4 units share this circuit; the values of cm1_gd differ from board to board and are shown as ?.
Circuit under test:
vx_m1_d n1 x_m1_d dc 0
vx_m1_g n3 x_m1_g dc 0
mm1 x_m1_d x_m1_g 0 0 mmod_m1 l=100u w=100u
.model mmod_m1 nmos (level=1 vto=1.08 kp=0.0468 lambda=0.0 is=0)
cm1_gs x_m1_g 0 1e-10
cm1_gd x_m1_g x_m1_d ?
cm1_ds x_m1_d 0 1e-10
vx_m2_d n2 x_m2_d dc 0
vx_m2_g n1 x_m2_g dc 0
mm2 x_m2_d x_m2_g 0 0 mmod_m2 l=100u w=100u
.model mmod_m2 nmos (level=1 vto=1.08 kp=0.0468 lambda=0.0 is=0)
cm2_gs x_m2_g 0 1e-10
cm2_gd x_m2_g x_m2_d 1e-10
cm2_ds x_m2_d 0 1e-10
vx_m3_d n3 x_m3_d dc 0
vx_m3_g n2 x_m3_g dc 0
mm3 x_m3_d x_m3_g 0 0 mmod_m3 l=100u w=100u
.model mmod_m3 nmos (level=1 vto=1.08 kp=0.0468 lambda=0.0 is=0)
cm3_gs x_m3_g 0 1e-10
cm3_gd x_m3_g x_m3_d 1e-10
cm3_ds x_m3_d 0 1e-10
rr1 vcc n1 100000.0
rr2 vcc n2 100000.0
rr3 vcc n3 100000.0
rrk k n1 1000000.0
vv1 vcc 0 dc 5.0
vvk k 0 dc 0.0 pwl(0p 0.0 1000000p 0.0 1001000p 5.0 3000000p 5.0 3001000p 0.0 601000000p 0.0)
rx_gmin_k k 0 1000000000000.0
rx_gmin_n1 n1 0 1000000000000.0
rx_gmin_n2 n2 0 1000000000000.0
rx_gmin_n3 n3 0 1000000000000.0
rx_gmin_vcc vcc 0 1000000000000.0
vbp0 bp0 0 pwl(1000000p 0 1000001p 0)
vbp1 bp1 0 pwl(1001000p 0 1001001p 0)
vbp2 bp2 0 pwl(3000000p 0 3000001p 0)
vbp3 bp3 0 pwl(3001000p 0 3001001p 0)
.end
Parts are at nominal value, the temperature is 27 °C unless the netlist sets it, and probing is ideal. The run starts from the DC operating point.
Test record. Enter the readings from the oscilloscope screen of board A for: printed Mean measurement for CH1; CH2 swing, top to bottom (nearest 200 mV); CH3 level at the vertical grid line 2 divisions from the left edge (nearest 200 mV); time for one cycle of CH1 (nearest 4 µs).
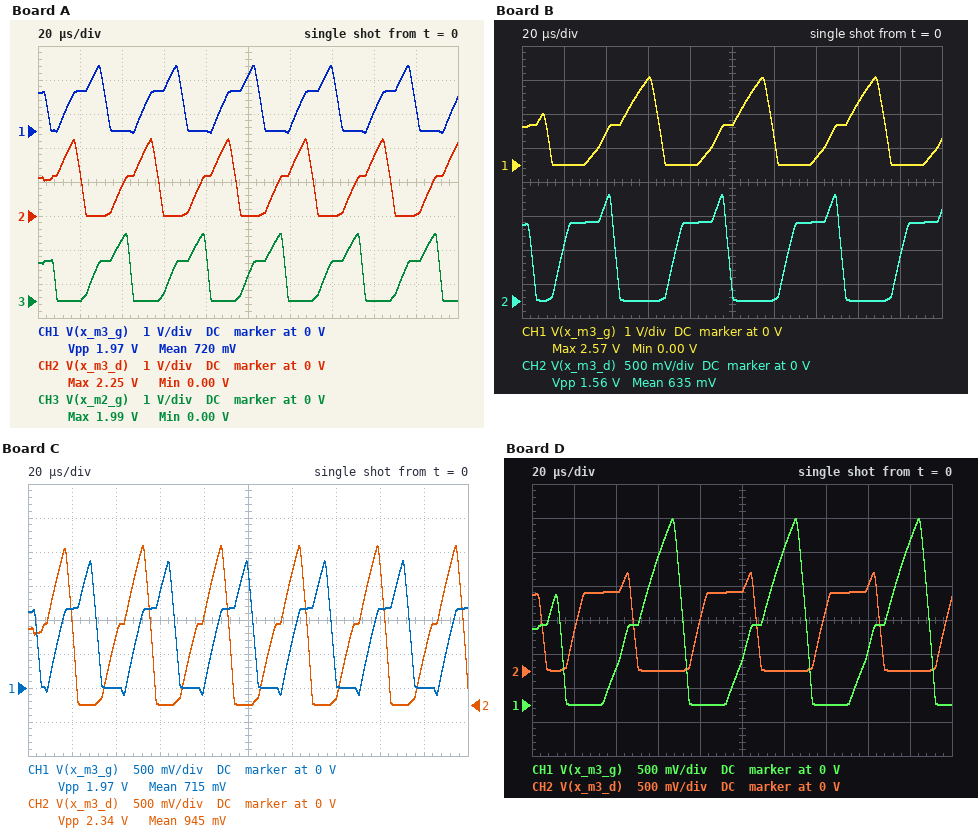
720 mV
2.2 V
1.8 V
36 µs
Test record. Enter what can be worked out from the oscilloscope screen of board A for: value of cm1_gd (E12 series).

56 pF
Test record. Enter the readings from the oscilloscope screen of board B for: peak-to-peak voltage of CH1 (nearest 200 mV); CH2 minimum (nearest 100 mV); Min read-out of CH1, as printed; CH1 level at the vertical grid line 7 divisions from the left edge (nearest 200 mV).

2.6 V
0 V
0.00 V
200 mV
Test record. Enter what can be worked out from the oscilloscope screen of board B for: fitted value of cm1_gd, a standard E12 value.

270 pF
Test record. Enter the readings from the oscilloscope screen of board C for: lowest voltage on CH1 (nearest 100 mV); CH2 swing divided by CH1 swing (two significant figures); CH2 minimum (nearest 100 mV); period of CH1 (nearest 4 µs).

-100 mV
1.2
0 V
36 µs
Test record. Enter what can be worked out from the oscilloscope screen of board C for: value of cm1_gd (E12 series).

39 pF
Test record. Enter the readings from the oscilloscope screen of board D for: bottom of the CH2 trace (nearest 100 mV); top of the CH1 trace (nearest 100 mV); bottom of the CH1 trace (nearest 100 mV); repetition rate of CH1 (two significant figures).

0 V
2.7 V
0 V
17 kHz
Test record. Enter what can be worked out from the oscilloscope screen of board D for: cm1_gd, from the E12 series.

330 pF
